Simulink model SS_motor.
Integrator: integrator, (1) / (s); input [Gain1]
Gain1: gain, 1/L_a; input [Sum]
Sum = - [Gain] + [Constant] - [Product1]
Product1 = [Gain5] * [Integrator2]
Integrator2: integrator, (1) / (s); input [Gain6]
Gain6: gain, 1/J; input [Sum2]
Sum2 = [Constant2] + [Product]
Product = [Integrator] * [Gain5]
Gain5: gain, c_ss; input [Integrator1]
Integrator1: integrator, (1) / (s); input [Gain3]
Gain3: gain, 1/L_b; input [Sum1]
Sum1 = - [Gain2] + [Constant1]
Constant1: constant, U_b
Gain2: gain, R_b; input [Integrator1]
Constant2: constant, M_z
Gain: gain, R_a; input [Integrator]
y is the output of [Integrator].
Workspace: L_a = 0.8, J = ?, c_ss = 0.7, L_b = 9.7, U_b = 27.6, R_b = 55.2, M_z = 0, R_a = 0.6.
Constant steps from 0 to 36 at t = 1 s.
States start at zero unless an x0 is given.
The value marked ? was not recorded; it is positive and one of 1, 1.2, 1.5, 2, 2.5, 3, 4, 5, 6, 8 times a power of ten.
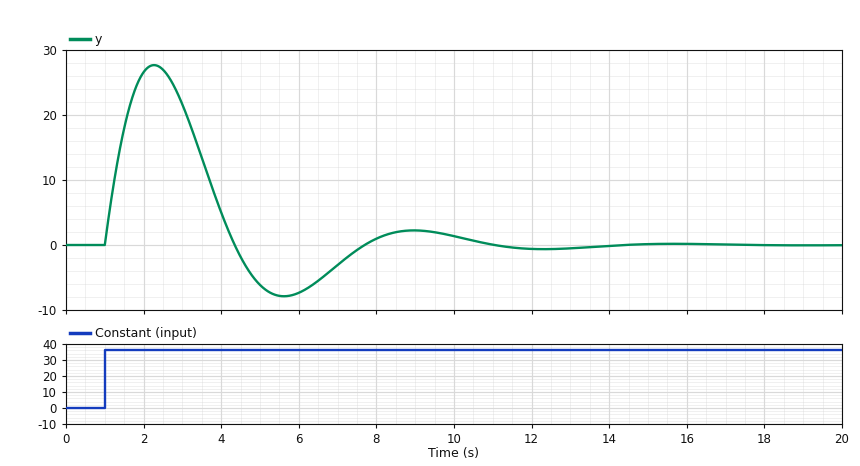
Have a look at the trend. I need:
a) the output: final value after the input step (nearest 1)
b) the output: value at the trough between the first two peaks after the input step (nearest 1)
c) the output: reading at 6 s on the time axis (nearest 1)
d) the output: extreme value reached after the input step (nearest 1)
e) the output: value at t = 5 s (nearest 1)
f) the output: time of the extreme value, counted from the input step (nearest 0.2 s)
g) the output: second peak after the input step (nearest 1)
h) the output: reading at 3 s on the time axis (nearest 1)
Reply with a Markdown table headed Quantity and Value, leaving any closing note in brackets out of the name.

| Quantity | Value |
|---|---|
| the output: final value after the input step | 0 |
| the output: value at the trough between the first two peaks after the input step | -8 |
| the output: reading at 6 s on the time axis | -7 |
| the output: extreme value reached after the input step | 28 |
| the output: value at t = 5 s | -6 |
| the output: time of the extreme value, counted from the input step | 1.2 s |
| the output: second peak after the input step | 2 |
| the output: reading at 3 s on the time axis | 22 |
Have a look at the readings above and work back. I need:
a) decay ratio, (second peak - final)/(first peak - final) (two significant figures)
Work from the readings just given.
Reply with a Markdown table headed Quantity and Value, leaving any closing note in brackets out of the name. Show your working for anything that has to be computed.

| Quantity | Value |
|---|---|
| decay ratio, (second peak - final)/(first peak - final) | (2 - 0) / (28 - 0) = 0.071 |
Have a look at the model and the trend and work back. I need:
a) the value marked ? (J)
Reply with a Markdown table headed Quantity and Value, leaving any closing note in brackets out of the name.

| Quantity | Value |
|---|---|
| the value marked ? | 0.15 |
